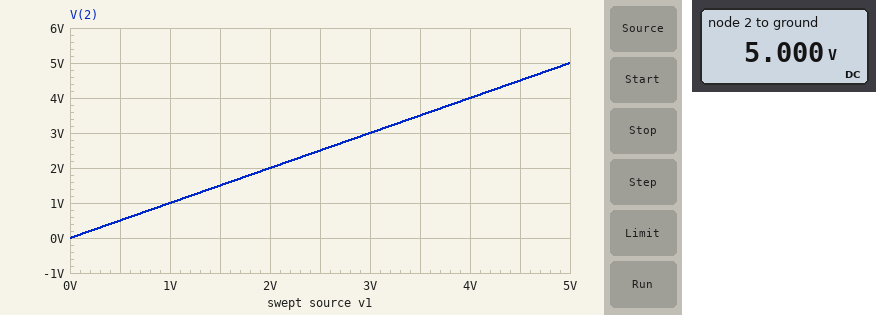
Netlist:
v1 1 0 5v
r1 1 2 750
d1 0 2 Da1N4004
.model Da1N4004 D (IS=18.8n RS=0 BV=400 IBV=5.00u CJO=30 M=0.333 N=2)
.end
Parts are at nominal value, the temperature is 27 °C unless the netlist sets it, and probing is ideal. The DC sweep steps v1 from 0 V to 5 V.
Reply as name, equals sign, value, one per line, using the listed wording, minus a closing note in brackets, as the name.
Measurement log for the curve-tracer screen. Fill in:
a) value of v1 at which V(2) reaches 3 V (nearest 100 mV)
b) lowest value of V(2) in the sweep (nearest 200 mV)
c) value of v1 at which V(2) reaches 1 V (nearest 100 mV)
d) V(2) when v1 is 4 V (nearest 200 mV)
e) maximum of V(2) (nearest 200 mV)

value of v1 at which V(2) reaches 3 V = 3.0 V
lowest value of V(2) in the sweep = 0 V
value of v1 at which V(2) reaches 1 V = 1.0 V
V(2) when v1 is 4 V = 4.0 V
maximum of V(2) = 5.0 V
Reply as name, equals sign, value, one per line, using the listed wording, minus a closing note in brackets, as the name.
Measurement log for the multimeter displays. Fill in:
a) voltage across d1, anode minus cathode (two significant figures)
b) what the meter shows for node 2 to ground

voltage across d1, anode minus cathode = -5.0 V
what the meter shows for node 2 to ground = 5.000 V
